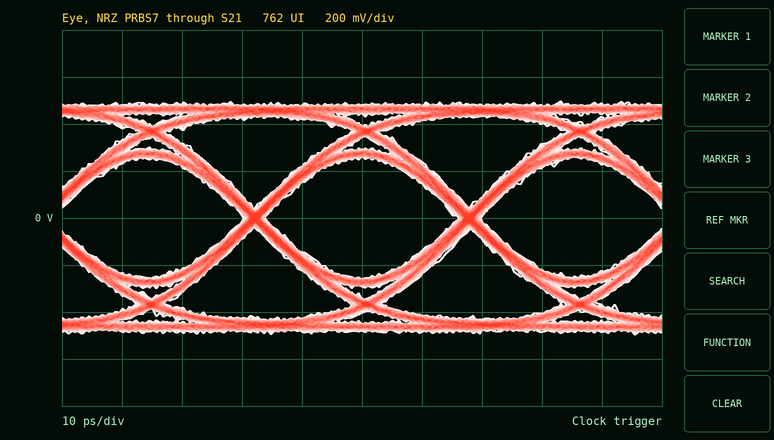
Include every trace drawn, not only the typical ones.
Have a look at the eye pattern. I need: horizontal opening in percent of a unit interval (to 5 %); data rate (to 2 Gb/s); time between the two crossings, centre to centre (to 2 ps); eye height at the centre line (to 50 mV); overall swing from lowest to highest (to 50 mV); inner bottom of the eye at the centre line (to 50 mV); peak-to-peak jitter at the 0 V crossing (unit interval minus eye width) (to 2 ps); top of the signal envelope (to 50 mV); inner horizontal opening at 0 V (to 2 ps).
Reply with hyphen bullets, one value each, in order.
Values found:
- 90 %
- 28 Gb/s
- 36 ps
- 500 mV
- 1.00 V
- -250 mV
- 4 ps
- 500 mV
- 32 ps
